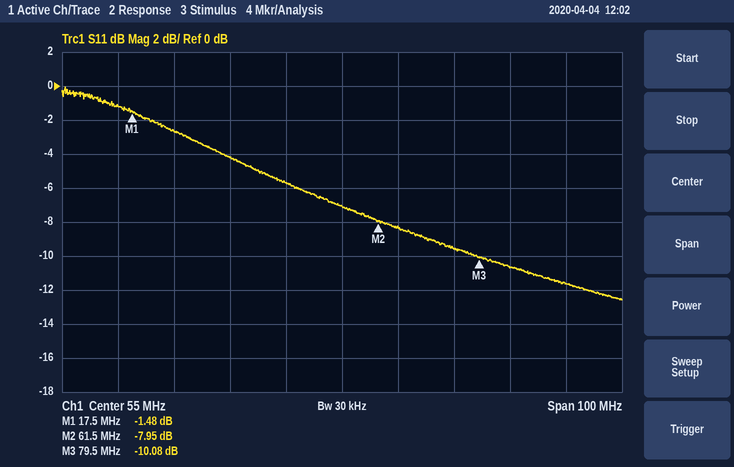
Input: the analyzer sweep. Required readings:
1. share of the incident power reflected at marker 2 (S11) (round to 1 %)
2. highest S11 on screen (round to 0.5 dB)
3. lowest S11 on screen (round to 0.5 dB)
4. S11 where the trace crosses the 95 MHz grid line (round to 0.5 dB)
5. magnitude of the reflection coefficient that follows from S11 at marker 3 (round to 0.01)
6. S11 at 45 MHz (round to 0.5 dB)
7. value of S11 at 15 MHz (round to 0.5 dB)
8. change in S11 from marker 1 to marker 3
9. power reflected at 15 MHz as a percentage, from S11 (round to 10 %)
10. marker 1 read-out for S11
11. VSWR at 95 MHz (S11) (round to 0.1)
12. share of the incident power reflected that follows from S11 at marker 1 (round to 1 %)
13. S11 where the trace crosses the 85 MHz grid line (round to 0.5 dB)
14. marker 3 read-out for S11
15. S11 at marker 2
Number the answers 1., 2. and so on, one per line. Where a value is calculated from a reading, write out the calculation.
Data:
1. 10^(-7.95/10) ≈ 16 %
2. 0.0 dB
3. -12.5 dB
4. -11.5 dB
5. 10^(-10.08/20) ≈ 0.31
6. -5.5 dB
7. -1.0 dB
8. -10.08 − (-1.48) = -8.60 dB
9. 10^(-1/10) ≈ 79.4 %, so 80 % to the nearest 10 %
10. -1.48 dB
11. |Γ| = 10^(-11.5/20) = 0.2661; VSWR = (1 + 0.2661)/(1 − 0.2661) ≈ 1.7
12. 10^(-1.48/10) ≈ 71 %
13. -10.5 dB
14. -10.08 dB
15. -7.95 dB
